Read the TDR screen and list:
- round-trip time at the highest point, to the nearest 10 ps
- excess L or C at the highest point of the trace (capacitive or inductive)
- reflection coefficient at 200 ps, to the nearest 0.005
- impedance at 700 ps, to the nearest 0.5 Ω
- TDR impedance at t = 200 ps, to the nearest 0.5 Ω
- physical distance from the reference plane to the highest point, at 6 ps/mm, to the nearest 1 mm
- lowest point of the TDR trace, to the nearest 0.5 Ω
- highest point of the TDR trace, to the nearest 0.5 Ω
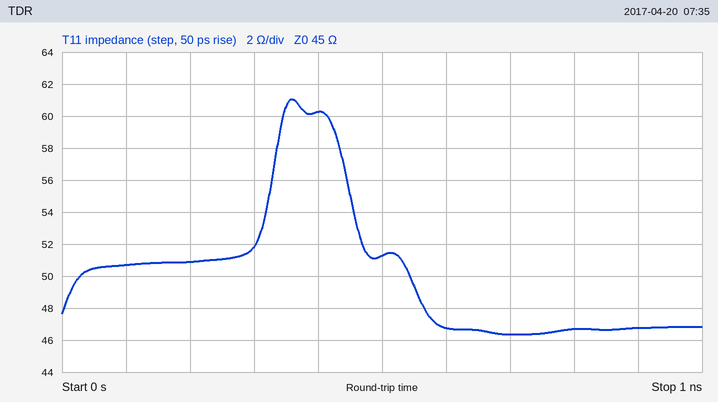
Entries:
360 ps
inductive
+0.060
46.5 Ω
51.0 Ω
30 mm
46.5 Ω
61.0 Ω
